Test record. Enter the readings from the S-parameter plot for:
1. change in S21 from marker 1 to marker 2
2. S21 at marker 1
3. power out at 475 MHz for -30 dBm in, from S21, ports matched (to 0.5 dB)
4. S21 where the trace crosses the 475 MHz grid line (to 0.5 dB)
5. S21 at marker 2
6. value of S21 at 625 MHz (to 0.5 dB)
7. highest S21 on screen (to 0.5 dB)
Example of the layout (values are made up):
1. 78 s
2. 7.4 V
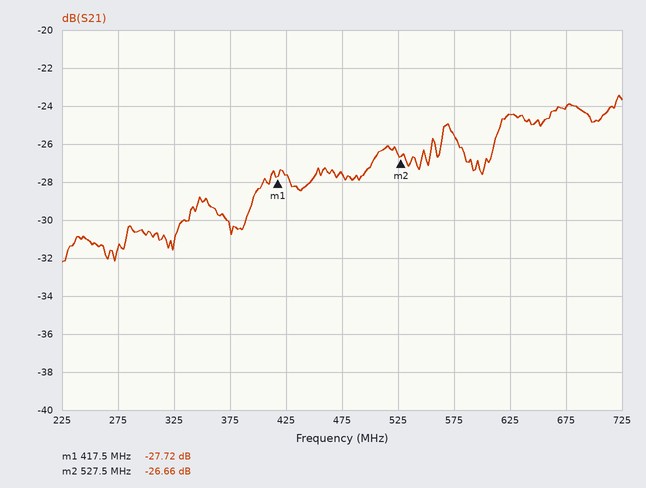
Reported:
1. 1.06 dB
2. -27.72 dB
3. -57.5 dBm
4. -27.5 dB
5. -26.66 dB
6. -24.5 dB
7. -23.5 dB
